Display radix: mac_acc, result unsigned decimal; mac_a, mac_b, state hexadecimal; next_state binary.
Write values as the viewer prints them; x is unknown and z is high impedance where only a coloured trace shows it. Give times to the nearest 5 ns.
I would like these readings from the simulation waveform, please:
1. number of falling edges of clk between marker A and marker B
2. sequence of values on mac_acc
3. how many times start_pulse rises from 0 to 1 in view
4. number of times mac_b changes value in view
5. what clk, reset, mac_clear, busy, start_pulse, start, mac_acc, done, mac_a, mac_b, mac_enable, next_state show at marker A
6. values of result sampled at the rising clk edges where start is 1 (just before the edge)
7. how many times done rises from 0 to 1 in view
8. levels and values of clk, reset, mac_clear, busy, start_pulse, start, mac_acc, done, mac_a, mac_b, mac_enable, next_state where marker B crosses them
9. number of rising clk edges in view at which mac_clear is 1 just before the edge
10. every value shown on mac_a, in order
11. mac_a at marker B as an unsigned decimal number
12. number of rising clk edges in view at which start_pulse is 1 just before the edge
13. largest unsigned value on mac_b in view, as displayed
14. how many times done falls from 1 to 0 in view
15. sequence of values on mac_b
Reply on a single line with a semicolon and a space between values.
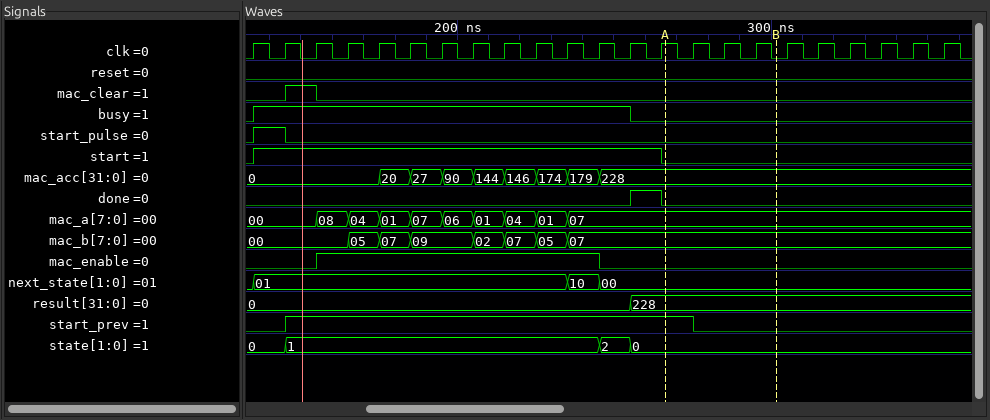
4; 0, 20, 27, 90, 144, 146, 174, 179, 228; 1; 7; clk=1, reset=0, mac_clear=0, busy=0, start_pulse=0, start=0, mac_acc=228, done=0, mac_a=07, mac_b=07, mac_enable=0, next_state=00; 0, 0, 0, 0, 0, 0, 0, 0, 0, 0, 0, 0, 228; 1; clk=0, reset=0, mac_clear=0, busy=0, start_pulse=0, start=0, mac_acc=228, done=0, mac_a=07, mac_b=07, mac_enable=0, next_state=00; 1; 00, 08, 04, 01, 07, 06, 01, 04, 01, 07; 7; 1; 09; 1; 00, 05, 07, 09, 02, 07, 05, 07
